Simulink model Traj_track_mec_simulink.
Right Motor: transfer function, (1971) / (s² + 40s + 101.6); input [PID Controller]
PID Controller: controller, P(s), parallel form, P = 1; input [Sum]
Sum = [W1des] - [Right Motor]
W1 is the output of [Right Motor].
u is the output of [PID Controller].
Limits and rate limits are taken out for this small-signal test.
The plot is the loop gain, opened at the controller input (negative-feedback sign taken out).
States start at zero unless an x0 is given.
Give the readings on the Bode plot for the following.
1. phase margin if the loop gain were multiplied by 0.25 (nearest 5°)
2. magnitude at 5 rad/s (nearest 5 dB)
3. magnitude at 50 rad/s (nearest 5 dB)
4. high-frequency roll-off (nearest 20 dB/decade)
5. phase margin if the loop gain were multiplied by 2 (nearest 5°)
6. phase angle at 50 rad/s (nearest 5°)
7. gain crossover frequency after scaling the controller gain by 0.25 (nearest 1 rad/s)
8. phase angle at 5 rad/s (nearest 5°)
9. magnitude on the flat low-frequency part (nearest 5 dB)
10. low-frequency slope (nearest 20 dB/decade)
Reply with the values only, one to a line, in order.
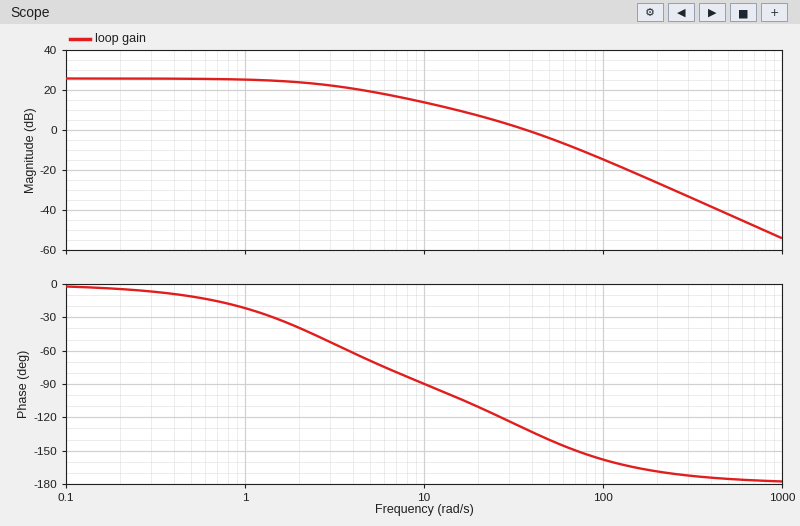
85°
20 dB
-5 dB
-40 dB/decade
35°
-140°
12 rad/s
-70°
25 dB
0 dB/decade
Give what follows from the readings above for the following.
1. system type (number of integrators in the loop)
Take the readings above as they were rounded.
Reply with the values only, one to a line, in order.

0
